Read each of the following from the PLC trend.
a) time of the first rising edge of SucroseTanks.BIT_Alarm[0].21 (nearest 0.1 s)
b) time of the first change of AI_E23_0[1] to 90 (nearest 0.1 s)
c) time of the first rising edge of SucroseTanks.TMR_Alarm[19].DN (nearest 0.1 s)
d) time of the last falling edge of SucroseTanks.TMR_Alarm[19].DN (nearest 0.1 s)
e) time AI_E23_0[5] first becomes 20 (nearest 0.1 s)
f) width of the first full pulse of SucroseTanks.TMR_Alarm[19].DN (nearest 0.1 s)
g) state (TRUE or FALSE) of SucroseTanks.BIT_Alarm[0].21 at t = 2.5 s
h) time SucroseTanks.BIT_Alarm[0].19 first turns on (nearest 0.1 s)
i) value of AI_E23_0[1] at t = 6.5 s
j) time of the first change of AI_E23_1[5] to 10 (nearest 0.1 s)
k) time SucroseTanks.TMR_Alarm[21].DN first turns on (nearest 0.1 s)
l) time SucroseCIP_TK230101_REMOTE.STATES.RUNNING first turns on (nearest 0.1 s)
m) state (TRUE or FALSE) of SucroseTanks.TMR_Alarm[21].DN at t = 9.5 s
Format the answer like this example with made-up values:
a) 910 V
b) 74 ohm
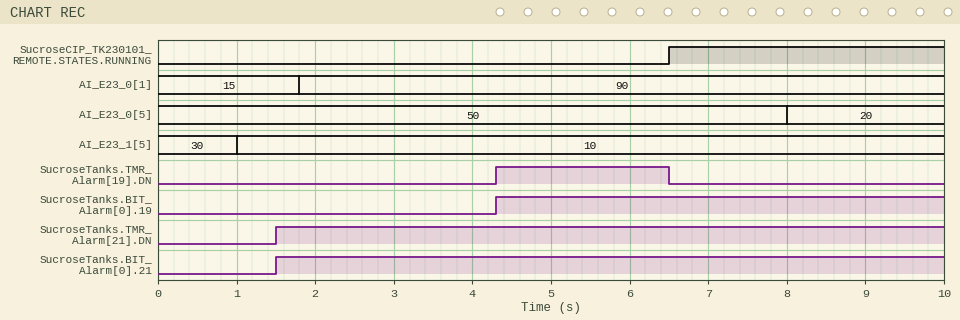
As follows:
a) 1.5 s
b) 1.8 s
c) 4.3 s
d) 6.5 s
e) 8.0 s
f) 2.2 s
g) TRUE
h) 4.3 s
i) 90
j) 1.0 s
k) 1.5 s
l) 6.5 s
m) TRUE
